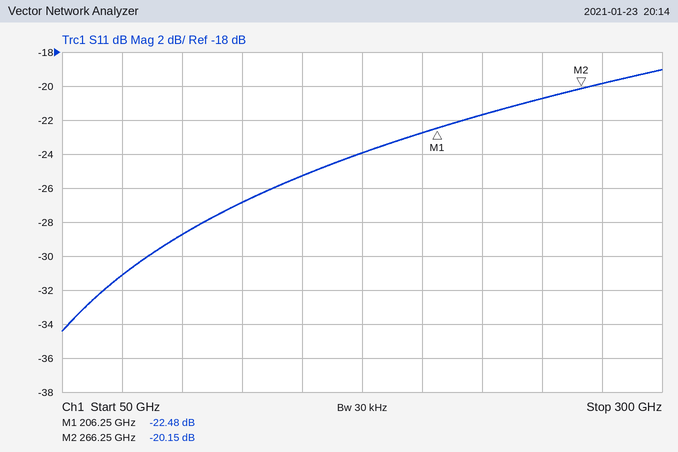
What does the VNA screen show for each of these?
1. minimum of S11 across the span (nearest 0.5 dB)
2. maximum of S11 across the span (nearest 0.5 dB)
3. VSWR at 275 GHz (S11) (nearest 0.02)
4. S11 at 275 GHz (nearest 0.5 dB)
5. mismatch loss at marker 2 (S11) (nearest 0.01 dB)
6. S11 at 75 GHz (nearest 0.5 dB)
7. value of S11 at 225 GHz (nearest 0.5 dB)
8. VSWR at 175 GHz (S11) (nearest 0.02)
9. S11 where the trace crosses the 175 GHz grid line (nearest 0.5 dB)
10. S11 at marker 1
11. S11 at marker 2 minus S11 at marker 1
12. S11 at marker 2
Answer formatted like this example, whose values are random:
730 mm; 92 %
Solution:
-34.5 dB; -19.0 dB; 1.22; -20.0 dB; 0.04 dB; -31.0 dB; -21.5 dB; 1.14; -24.0 dB; -22.48 dB; 2.33 dB; -20.15 dB
